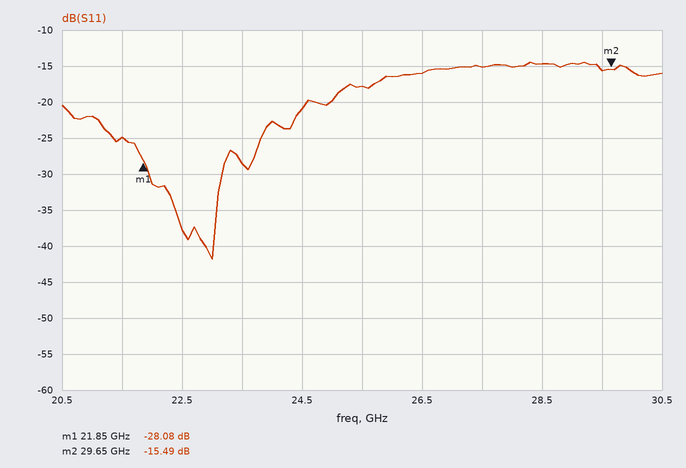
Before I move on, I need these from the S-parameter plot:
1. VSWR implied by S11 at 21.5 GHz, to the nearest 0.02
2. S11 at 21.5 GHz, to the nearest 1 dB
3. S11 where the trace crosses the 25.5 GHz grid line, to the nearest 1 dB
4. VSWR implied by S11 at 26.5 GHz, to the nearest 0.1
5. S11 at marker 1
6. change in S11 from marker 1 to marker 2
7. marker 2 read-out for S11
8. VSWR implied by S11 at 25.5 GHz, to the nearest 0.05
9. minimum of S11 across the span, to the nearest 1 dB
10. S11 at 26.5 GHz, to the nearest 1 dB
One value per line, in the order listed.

1.12
-25 dB
-18 dB
1.4
-28.08 dB
12.59 dB
-15.49 dB
1.30
-42 dB
-16 dB
